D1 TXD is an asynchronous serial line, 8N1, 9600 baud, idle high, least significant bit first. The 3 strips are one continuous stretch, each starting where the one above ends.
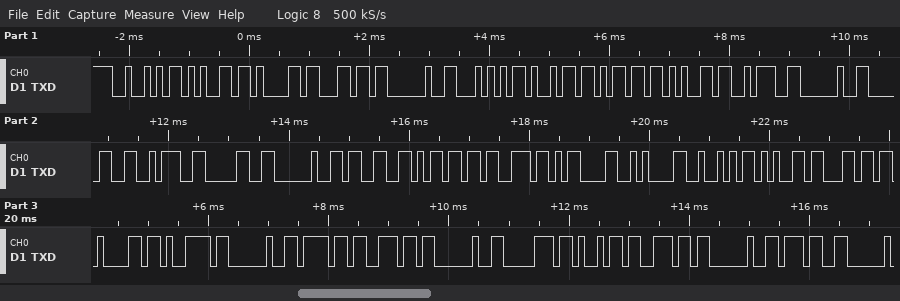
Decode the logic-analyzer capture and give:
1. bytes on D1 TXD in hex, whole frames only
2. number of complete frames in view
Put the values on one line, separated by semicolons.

0x52 0x65 0x61 0x6C 0x20 0x54 0x69 0x6D 0x65 0x3A 0x20 0x30 0x3A 0x30 0x20 0x33 0x6D 0x73 0x0D 0x0A 0x52 0x65 0x6C 0x61 0x79 0x20 0x6F 0x6E 0x20 0x70 0x69 0x6E 0x20 0x37; 34
